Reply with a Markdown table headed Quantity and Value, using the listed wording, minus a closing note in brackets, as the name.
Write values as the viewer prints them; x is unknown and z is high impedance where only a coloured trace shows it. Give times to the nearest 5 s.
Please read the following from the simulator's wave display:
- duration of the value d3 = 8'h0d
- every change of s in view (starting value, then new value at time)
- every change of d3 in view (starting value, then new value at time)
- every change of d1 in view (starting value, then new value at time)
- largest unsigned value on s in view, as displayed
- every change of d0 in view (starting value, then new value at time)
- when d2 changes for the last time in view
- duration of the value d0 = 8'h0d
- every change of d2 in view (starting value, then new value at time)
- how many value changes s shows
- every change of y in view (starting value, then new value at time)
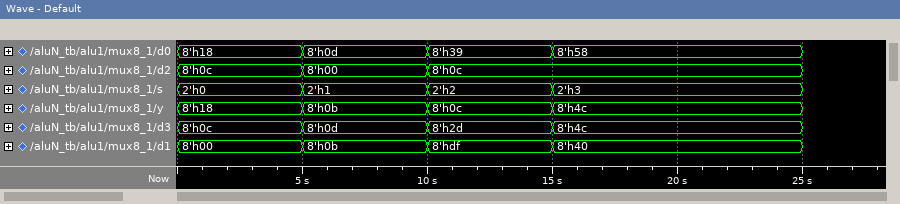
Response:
| Quantity | Value |
|---|---|
| duration of the value d3 = 8'h0d | 5 s |
| every change of s in view | 2'h0, 2'h1 at 5 s, 2'h2 at 10 s, 2'h3 at 15 s |
| every change of d3 in view | 8'h0c, 8'h0d at 5 s, 8'h2d at 10 s, 8'h4c at 15 s |
| every change of d1 in view | 8'h00, 8'h0b at 5 s, 8'hdf at 10 s, 8'h40 at 15 s |
| largest unsigned value on s in view, as displayed | 2'h3 |
| every change of d0 in view | 8'h18, 8'h0d at 5 s, 8'h39 at 10 s, 8'h58 at 15 s |
| when d2 changes for the last time in view | 10 s |
| duration of the value d0 = 8'h0d | 5 s |
| every change of d2 in view | 8'h0c, 8'h00 at 5 s, 8'h0c at 10 s |
| how many value changes s shows | 3 |
| every change of y in view | 8'h18, 8'h0b at 5 s, 8'h0c at 10 s, 8'h4c at 15 s |
